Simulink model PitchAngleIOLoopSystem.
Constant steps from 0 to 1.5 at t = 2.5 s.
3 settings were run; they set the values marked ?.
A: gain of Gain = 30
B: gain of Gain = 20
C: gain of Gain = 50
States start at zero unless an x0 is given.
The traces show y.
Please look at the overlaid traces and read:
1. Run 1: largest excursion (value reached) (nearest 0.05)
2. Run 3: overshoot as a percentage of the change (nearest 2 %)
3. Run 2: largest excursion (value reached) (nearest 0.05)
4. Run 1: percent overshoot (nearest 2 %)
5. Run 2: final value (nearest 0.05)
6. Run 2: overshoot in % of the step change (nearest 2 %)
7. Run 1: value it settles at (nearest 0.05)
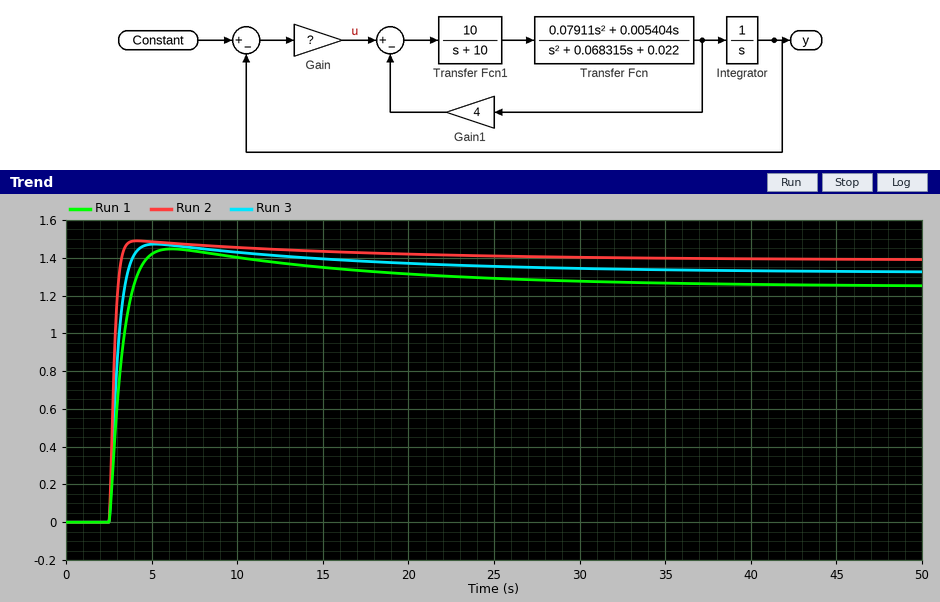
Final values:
1.45
12 %
1.50
16 %
1.40
8 %
1.25
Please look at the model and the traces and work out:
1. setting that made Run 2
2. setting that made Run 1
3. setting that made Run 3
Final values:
C
B
A
